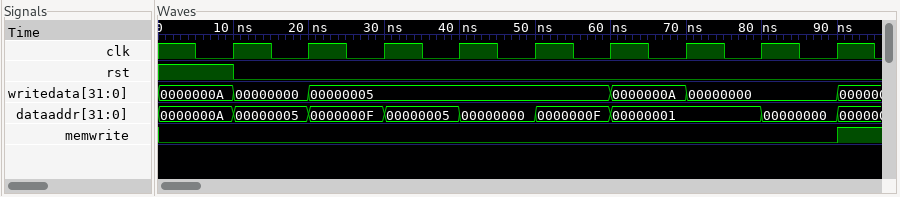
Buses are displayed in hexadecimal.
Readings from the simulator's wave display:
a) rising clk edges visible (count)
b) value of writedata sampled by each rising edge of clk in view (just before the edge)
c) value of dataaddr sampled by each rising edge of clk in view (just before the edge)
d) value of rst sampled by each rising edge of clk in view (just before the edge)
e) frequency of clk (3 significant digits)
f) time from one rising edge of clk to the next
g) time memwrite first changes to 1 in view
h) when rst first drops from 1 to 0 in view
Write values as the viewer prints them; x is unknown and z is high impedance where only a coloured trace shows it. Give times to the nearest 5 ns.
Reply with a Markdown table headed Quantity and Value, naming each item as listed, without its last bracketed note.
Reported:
| Quantity | Value |
|---|---|
| rising clk edges visible | 9 |
| value of writedata sampled by each rising edge of clk in view | 0000000A, 00000000, 00000005, 00000005, 00000005, 00000005, 0000000A, 00000000, 00000000 |
| value of dataaddr sampled by each rising edge of clk in view | 0000000A, 00000005, 0000000F, 00000005, 00000000, 0000000F, 00000001, 00000001, 00000000 |
| value of rst sampled by each rising edge of clk in view | 1 0 0 0 0 0 0 0 0 |
| frequency of clk | 100 MHz |
| time from one rising edge of clk to the next | 10 ns |
| time memwrite first changes to 1 in view | 90 ns |
| when rst first drops from 1 to 0 in view | 10 ns |
